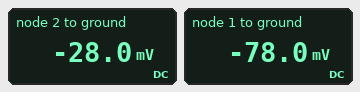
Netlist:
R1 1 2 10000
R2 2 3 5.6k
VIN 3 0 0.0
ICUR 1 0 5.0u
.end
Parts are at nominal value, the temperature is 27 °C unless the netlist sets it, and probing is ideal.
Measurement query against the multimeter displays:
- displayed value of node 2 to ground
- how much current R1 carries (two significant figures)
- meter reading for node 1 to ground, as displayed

-28.0 mV
5.0 µA
-78.0 mV
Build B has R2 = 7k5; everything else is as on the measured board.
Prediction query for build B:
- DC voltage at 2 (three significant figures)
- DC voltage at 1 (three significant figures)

-37.5 mV
-87.5 mV
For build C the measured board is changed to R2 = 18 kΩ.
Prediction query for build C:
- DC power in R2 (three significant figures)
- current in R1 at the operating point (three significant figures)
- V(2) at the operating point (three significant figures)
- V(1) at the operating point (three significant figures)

450 nW
5.00 µA
-90.0 mV
-140 mV
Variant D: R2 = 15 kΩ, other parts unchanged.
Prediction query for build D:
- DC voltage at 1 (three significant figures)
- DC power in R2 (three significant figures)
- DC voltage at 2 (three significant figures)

-125 mV
375 nW
-75.0 mV
